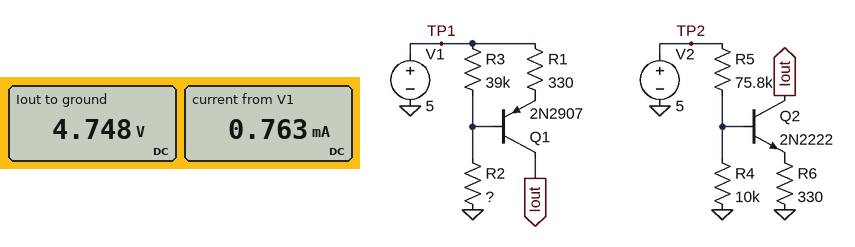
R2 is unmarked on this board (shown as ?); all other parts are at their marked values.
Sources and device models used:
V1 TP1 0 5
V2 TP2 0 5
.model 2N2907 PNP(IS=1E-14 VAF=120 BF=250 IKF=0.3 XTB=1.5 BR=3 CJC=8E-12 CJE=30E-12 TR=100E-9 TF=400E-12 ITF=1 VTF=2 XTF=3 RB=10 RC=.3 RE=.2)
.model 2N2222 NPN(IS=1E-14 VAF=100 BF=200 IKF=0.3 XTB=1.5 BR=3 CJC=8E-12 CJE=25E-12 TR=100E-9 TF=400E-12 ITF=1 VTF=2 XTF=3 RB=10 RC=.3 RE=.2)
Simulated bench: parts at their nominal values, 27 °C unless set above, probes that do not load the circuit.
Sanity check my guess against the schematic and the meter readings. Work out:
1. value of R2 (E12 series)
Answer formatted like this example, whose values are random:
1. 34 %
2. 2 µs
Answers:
1. 5.6 kΩ
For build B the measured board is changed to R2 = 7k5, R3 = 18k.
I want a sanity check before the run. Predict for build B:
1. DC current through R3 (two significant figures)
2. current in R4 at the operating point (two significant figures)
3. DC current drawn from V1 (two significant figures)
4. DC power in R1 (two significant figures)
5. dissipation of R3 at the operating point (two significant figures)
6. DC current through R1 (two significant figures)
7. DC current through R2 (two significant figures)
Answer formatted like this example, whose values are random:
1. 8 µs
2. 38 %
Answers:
1. 48 µA
2. 58 µA
3. 590 µA
4. 97 µW
5. 41 µW
6. 540 µA
7. 550 µA
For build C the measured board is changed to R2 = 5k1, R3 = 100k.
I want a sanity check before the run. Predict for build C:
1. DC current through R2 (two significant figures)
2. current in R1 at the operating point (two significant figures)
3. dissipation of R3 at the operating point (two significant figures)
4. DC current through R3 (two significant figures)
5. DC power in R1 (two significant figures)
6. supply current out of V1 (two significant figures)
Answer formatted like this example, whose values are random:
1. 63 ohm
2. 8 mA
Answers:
1. 790 µA
2. 820 µA
3. 9.3 µW
4. 9.6 µA
5. 220 µW
6. 830 µA
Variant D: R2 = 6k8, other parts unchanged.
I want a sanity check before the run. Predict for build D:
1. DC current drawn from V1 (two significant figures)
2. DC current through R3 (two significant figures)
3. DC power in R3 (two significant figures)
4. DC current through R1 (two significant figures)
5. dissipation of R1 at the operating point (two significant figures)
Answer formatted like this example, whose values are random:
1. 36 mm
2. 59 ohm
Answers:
1. 640 µA
2. 23 µA
3. 20 µW
4. 620 µA
5. 130 µW
